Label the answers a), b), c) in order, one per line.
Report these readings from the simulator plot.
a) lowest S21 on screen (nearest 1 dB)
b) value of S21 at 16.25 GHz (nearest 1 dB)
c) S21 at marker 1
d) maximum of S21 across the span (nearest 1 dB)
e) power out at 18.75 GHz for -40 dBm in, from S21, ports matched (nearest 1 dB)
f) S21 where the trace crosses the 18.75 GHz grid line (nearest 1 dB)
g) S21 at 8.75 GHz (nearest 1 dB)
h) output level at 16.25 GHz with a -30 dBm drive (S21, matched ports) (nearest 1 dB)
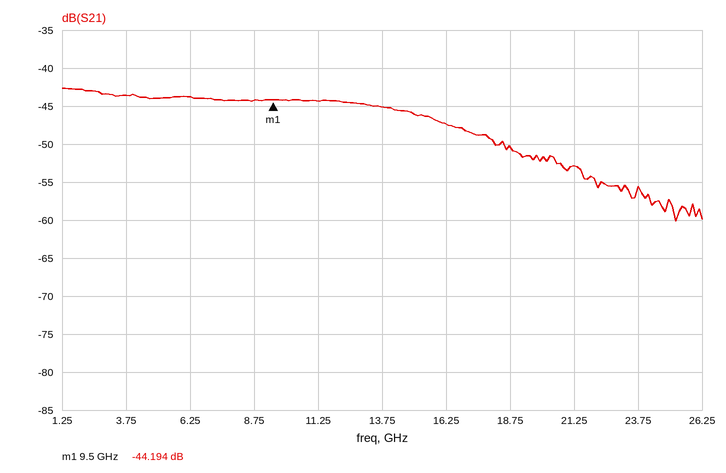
a) -60 dB
b) -47 dB
c) -44.194 dB
d) -43 dB
e) -90 dBm
f) -50 dB
g) -44 dB
h) -77 dBm
